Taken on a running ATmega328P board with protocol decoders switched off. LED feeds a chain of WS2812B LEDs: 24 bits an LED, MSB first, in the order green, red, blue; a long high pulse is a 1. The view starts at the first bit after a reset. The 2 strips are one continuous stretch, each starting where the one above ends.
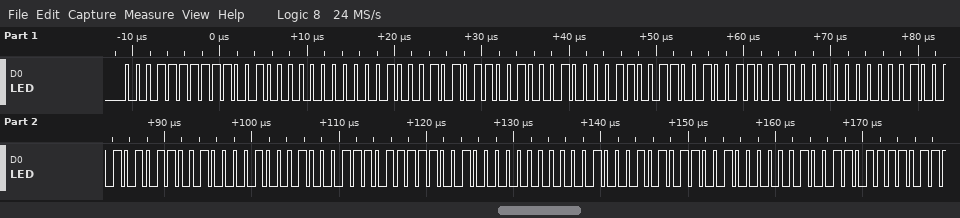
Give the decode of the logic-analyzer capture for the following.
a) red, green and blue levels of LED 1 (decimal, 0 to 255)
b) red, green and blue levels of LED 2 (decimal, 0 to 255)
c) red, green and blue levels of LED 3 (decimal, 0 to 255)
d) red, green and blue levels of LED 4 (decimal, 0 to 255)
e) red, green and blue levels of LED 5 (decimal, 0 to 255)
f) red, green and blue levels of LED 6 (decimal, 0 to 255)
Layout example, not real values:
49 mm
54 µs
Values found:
200, 31, 0
200, 138, 134
200, 100, 0
200, 138, 68
200, 119, 0
200, 138, 19
